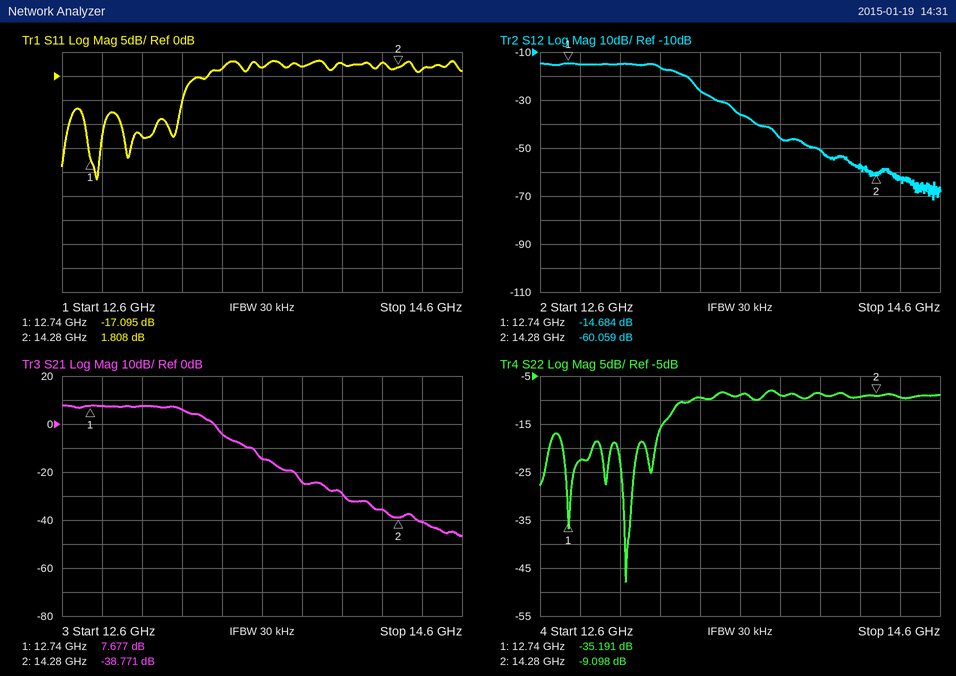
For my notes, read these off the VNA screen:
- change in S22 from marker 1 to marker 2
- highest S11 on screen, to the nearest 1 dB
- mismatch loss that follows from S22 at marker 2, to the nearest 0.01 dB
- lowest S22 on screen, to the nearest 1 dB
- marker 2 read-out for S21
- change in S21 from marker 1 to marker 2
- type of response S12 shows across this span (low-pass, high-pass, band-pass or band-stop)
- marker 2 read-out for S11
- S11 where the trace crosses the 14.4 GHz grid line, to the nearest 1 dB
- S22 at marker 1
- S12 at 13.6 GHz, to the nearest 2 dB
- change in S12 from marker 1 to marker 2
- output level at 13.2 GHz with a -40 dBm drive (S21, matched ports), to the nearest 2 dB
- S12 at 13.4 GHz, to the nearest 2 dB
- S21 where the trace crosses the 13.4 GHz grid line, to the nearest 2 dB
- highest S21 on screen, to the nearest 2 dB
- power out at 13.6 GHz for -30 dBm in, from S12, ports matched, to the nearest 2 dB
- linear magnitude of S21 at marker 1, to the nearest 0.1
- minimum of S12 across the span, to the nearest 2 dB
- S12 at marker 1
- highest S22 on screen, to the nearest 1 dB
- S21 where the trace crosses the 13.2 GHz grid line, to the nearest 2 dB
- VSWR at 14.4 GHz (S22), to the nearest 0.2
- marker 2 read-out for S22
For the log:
26.093 dB
3 dB
0.57 dB
-48 dB
-38.771 dB
-46.448 dB
low-pass
1.808 dB
1 dB
-35.191 dB
-36 dB
-45.375 dB
-34 dBm
-26 dB
-4 dB
8 dB
-66 dBm
2.4
-72 dB
-14.684 dB
-8 dB
6 dB
2.0
-9.098 dB
